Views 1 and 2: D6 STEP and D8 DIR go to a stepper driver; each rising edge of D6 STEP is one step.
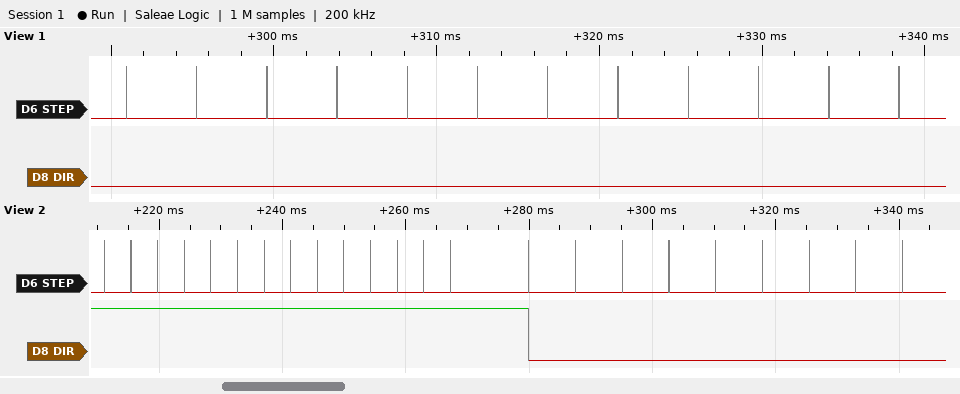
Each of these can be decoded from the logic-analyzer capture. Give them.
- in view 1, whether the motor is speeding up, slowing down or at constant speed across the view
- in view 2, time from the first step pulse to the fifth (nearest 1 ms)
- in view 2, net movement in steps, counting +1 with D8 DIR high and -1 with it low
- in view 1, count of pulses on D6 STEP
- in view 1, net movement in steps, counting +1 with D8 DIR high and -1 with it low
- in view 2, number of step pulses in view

constant speed
17 ms
+5
12
-12
23
